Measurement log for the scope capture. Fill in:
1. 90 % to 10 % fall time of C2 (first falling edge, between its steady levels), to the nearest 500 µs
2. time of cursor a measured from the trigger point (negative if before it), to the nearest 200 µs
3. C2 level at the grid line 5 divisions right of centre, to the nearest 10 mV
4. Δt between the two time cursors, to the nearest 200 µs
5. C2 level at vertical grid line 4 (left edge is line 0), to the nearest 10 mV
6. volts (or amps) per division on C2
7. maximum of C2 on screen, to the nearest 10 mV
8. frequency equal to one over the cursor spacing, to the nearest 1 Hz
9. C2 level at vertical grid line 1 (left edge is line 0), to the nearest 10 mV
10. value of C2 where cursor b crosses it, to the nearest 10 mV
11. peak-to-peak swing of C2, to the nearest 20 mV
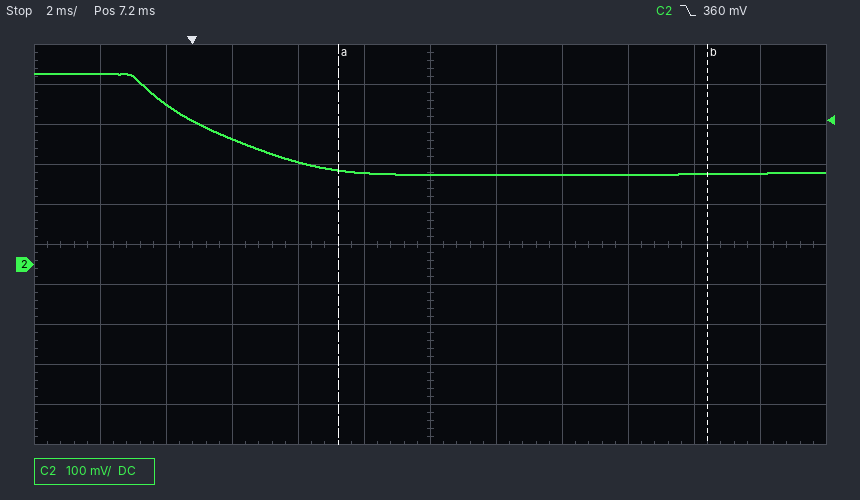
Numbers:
5.0 ms
+4.4 ms
230 mV
11.2 ms
260 mV
100 mV
480 mV
89 Hz
480 mV
230 mV
260 mV
